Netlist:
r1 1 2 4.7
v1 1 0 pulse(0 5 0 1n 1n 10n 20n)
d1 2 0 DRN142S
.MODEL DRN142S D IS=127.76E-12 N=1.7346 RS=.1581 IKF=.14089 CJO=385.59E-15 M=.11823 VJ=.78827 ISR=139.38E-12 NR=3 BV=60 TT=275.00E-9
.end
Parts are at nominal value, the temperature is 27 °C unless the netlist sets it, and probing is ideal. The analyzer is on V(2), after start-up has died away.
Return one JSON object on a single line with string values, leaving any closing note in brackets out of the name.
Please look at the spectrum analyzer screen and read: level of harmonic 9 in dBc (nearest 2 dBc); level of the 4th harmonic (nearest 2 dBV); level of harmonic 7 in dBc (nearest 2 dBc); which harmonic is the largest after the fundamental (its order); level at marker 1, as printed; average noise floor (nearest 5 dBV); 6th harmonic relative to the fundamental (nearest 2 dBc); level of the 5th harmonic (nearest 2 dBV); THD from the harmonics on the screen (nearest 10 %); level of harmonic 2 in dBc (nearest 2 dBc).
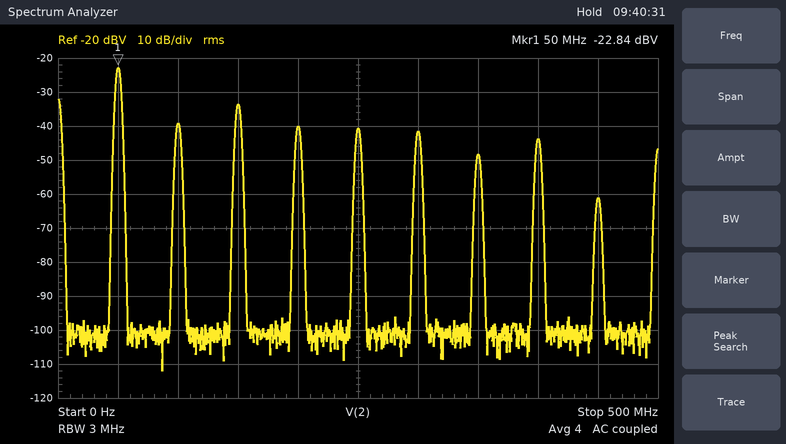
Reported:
{"level of harmonic 9 in dBc": "-38 dBc", "level of the 4th harmonic": "-40 dBV", "level of harmonic 7 in dBc": "-26 dBc", "which harmonic is the largest after the fundamental": "3", "level at marker 1, as printed": "-22.84 dBV", "average noise floor": "-100 dBV", "6th harmonic relative to the fundamental": "-18 dBc", "level of the 5th harmonic": "-40 dBV", "THD from the harmonics on the screen": "40 %", "level of harmonic 2 in dBc": "-16 dBc"}
